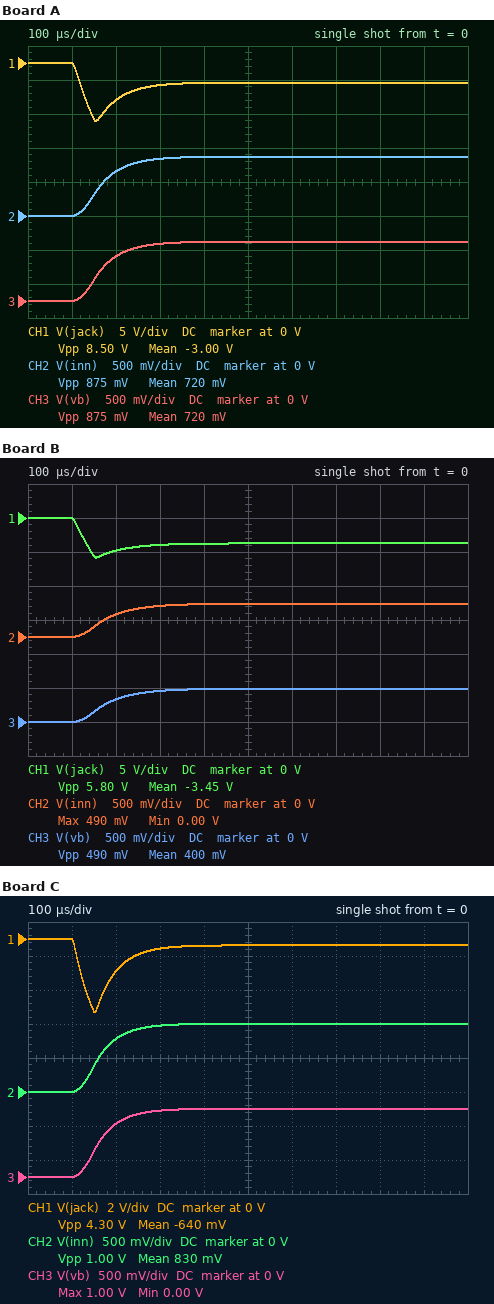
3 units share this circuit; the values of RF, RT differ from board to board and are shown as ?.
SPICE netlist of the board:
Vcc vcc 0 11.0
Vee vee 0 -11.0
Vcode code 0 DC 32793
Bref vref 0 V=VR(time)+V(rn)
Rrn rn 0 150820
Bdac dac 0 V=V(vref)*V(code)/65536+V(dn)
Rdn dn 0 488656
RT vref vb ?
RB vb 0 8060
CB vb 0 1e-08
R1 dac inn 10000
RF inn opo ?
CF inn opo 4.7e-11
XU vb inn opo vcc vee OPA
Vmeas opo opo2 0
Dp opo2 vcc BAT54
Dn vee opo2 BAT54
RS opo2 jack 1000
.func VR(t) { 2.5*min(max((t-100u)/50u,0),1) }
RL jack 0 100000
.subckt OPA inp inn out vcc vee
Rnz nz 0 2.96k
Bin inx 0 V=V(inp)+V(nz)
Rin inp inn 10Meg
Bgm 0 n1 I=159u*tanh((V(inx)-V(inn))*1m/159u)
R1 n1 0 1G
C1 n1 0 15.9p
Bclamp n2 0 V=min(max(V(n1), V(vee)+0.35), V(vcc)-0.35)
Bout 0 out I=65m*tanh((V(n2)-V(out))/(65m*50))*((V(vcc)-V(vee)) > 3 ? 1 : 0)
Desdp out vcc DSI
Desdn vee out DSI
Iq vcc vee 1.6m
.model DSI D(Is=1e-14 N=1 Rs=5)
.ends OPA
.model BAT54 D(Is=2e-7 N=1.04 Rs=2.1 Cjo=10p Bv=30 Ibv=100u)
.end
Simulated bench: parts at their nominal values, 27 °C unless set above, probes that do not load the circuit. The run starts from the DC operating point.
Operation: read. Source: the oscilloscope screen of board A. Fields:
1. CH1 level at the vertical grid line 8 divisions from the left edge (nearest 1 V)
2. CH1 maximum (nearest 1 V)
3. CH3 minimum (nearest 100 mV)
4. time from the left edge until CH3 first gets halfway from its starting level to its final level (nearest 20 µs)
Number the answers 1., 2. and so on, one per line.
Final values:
1. -3 V
2. 0 V
3. 0 V
4. 160 µs
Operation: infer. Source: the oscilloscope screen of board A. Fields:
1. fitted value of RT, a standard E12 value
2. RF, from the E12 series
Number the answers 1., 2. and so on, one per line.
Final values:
1. 15 kΩ
2. 100 kΩ
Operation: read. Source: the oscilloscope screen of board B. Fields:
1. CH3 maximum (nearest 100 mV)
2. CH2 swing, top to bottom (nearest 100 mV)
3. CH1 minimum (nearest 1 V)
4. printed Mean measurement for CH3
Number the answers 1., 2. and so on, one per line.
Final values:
1. 500 mV
2. 500 mV
3. -6 V
4. 400 mV
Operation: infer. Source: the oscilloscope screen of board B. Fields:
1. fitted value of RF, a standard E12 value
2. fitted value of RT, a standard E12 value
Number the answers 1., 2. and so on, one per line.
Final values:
1. 56 kΩ
2. 33 kΩ
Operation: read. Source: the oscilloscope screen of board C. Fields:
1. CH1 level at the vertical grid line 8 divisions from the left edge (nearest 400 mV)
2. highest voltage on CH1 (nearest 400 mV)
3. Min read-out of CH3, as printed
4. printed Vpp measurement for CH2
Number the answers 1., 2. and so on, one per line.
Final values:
1. -400 mV
2. 0 V
3. 0.00 V
4. 1.00 V
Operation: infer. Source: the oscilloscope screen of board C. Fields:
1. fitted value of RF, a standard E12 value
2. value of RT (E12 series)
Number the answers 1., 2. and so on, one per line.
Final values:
1. 56 kΩ
2. 12 kΩ
